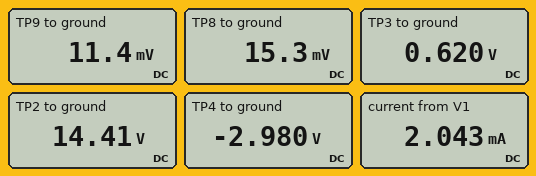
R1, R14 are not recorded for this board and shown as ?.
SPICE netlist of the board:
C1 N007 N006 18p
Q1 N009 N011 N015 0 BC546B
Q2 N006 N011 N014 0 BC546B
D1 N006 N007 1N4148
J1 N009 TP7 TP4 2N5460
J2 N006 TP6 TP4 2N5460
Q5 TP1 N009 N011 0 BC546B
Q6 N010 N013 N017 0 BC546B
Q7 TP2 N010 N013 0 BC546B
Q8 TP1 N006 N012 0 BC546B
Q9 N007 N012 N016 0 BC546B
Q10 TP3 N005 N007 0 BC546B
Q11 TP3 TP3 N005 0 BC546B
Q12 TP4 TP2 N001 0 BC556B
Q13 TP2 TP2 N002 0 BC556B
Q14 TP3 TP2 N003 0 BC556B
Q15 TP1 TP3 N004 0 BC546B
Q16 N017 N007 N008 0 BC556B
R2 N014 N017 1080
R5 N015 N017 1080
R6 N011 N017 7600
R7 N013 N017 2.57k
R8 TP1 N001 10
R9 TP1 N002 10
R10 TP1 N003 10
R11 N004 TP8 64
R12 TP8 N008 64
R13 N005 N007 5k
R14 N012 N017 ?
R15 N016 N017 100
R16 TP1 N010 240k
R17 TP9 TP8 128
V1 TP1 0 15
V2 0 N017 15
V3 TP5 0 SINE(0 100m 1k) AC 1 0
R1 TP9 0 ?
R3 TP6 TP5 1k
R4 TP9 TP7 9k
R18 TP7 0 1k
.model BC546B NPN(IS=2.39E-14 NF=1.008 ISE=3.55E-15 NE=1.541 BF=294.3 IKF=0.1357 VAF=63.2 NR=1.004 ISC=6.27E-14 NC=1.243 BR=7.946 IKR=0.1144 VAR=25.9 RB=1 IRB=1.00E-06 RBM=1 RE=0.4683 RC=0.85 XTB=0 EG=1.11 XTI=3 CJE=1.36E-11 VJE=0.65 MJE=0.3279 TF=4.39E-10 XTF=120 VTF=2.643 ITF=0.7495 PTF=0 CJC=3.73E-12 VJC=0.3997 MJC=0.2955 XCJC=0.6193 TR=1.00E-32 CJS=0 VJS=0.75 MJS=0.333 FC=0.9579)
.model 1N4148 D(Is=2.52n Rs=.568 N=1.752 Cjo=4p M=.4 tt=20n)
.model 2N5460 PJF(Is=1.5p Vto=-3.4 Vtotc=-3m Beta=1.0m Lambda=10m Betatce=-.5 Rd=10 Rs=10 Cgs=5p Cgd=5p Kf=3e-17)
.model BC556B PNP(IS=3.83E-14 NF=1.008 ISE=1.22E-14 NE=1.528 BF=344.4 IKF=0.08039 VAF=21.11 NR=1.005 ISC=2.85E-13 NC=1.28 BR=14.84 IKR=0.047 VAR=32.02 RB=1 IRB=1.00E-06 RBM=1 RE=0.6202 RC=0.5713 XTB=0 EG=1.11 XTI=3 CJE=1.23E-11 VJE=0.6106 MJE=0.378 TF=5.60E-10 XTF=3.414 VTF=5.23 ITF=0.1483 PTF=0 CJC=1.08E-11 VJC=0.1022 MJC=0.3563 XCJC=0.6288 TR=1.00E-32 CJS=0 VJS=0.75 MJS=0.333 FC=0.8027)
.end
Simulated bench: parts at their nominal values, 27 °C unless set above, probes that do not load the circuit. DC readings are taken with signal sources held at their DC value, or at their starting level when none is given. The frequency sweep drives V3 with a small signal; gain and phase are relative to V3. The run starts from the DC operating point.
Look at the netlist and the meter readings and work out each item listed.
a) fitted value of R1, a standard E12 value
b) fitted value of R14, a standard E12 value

390 Ω
1 kΩ
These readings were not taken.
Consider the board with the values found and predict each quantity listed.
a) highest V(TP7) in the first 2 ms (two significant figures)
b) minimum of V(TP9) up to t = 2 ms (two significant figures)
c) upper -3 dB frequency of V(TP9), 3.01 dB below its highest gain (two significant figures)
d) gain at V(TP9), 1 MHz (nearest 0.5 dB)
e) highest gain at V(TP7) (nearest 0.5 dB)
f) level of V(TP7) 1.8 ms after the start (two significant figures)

100 mV
-990 mV
490 kHz
13.0 dB
0 dB
-94 mV
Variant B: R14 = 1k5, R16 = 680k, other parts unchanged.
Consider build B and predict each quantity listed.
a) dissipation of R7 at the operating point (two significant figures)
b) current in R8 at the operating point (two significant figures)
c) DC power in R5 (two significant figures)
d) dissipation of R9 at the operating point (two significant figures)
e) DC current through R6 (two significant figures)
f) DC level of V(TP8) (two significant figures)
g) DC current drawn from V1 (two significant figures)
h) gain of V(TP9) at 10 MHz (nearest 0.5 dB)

120 µW
370 µA
37 µW
460 nW
100 µA
8.0 mV
1.7 mA
-5.0 dB
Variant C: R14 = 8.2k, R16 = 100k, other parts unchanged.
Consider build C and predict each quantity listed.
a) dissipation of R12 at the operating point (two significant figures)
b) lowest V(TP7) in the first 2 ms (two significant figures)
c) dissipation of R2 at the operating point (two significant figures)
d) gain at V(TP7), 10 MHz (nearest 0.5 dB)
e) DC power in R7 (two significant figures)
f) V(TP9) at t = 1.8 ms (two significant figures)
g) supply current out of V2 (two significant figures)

2.6 µW
-100 mV
44 µW
-18.0 dB
140 µW
-960 mV
1.7 mA
